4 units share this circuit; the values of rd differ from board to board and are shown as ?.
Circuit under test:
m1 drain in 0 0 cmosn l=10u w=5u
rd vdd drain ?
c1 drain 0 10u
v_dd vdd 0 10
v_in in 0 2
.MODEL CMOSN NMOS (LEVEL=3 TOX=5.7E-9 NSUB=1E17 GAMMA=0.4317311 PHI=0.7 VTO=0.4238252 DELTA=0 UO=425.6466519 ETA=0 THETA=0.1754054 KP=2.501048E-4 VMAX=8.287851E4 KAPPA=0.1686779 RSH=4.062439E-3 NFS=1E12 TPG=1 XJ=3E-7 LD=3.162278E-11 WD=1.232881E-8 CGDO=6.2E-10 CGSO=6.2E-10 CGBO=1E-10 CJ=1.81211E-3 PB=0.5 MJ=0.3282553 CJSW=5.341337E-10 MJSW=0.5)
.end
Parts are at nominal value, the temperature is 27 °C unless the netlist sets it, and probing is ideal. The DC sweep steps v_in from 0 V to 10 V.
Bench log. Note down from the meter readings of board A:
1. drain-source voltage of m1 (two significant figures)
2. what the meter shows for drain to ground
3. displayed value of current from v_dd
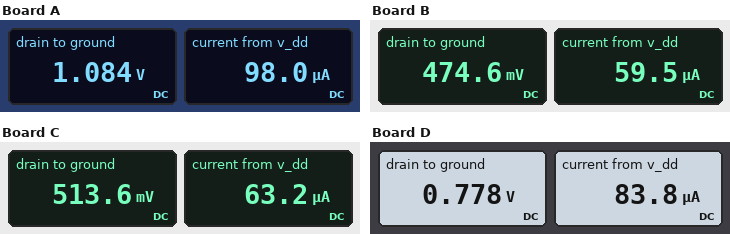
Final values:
1.1 V
1.084 V
98.0 µA
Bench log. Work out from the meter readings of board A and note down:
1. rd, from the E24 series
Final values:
91 kΩ
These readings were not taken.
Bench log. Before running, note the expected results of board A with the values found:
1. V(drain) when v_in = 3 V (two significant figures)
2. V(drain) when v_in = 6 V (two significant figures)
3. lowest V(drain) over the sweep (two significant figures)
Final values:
540 mV
320 mV
250 mV
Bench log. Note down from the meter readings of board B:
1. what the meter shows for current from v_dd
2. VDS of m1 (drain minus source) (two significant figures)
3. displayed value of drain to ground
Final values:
59.5 µA
470 mV
474.6 mV
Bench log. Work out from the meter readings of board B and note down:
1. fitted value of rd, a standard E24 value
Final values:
160 kΩ
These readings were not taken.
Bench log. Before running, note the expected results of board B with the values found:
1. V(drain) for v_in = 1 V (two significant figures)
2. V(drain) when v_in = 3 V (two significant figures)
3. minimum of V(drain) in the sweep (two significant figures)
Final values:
7.4 V
300 mV
140 mV
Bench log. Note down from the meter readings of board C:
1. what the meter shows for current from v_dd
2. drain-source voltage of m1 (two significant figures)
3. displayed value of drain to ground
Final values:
63.2 µA
510 mV
513.6 mV
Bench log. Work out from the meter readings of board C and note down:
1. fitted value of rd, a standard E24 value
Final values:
150 kΩ
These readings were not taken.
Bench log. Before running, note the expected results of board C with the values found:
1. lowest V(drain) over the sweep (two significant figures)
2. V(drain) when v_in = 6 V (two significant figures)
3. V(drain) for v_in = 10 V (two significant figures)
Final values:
150 mV
190 mV
150 mV
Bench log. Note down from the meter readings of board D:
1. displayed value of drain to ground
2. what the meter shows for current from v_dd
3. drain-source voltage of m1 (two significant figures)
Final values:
0.778 V
83.8 µA
780 mV
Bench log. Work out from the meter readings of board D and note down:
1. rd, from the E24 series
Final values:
110 kΩ
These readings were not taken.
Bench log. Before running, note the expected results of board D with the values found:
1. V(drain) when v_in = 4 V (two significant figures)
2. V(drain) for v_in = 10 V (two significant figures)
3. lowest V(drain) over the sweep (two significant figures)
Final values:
340 mV
200 mV
200 mV
